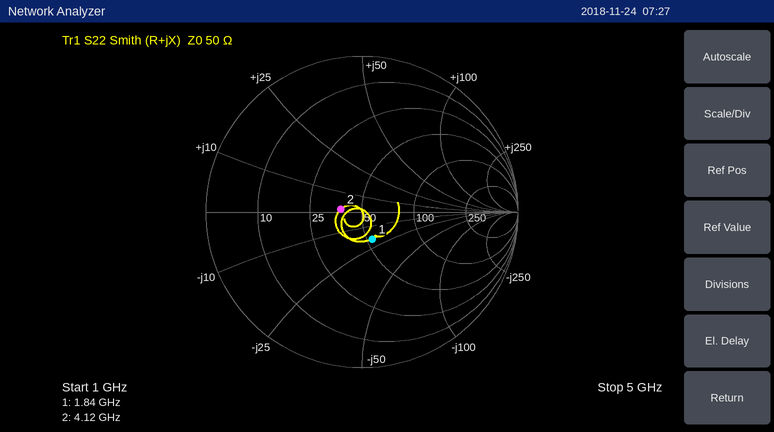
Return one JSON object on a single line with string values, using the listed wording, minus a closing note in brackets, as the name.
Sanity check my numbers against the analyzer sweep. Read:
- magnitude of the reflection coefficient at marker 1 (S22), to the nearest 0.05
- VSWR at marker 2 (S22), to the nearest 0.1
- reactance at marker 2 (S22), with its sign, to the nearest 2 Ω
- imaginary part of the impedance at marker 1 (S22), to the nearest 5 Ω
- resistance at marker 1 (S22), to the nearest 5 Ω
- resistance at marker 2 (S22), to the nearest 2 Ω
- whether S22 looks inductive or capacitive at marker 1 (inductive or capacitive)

{"magnitude of the reflection coefficient at marker 1 (S22), to the nearest 0.05": "0.20", "VSWR at marker 2 (S22), to the nearest 0.1": "1.3", "reactance at marker 2 (S22), with its sign, to the nearest 2 Ω": "+2 Ω", "imaginary part of the impedance at marker 1 (S22), to the nearest 5 Ω": "-20 Ω", "resistance at marker 1 (S22), to the nearest 5 Ω": "55 Ω", "resistance at marker 2 (S22), to the nearest 2 Ω": "38 Ω", "whether S22 looks inductive or capacitive at marker 1": "capacitive"}
